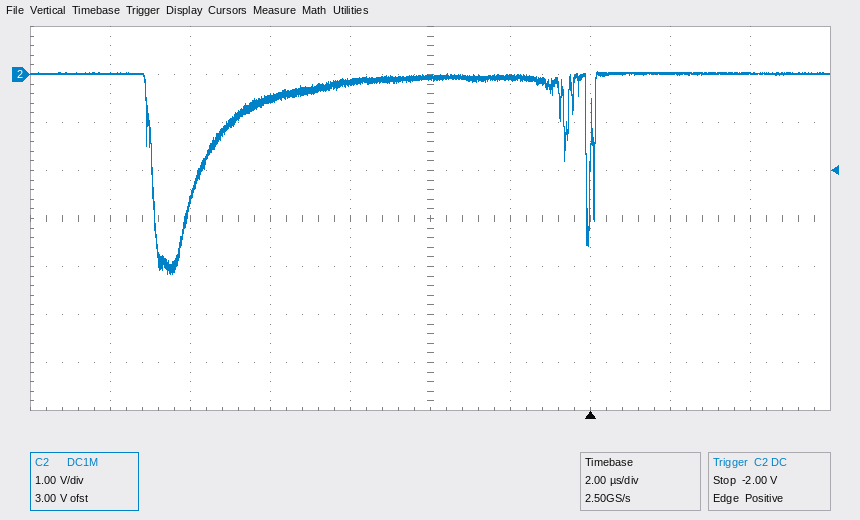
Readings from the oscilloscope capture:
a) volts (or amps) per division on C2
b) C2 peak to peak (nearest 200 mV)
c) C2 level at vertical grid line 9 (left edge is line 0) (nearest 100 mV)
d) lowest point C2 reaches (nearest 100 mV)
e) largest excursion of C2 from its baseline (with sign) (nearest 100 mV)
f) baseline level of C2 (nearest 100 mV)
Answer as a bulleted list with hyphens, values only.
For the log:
- 1 V
- 4.2 V
- 0.0 V
- -4.2 V
- -4.2 V
- 0.0 V
